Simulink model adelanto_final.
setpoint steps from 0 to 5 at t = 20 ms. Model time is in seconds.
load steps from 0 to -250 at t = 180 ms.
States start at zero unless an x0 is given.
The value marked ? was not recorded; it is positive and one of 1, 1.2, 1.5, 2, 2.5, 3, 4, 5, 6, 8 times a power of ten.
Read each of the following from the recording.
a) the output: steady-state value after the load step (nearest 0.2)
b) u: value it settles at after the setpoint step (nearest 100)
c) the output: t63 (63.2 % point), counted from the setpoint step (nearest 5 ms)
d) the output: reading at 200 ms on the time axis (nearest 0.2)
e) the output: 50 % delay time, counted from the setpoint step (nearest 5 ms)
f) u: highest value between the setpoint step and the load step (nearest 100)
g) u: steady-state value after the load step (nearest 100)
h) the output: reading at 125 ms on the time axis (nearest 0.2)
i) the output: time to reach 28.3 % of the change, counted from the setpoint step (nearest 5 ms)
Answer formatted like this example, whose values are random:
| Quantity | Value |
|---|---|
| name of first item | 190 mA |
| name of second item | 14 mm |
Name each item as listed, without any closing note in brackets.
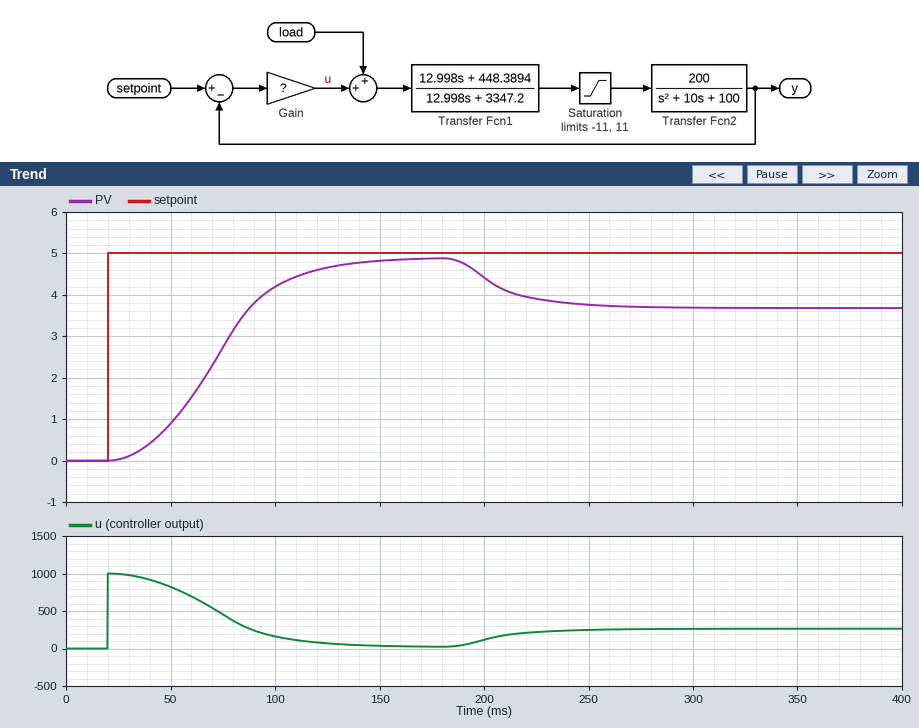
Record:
| Quantity | Value |
|---|---|
| the output: steady-state value after the load step | 3.6 |
| u: value it settles at after the setpoint step | 0 |
| the output: t63 (63.2 % point), counted from the setpoint step | 60 ms |
| the output: reading at 200 ms on the time axis | 4.4 |
| the output: 50 % delay time, counted from the setpoint step | 50 ms |
| u: highest value between the setpoint step and the load step | 1000 |
| u: steady-state value after the load step | 300 |
| the output: reading at 125 ms on the time axis | 4.6 |
| the output: time to reach 28.3 % of the change, counted from the setpoint step | 40 ms |
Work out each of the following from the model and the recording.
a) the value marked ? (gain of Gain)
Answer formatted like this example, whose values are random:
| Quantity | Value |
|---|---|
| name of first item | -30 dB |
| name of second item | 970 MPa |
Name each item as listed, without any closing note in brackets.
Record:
| Quantity | Value |
|---|---|
| the value marked ? | 200 |
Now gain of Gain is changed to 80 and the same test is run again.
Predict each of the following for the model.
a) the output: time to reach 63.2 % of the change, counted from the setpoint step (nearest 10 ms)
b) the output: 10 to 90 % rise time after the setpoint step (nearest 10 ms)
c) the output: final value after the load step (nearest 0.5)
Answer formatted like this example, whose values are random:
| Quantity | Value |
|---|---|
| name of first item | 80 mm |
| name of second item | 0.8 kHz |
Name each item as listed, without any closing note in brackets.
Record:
| Quantity | Value |
|---|---|
| the output: time to reach 63.2 % of the change, counted from the setpoint step | 60 ms |
| the output: 10 to 90 % rise time after the setpoint step | 60 ms |
| the output: final value after the load step | 2.0 |
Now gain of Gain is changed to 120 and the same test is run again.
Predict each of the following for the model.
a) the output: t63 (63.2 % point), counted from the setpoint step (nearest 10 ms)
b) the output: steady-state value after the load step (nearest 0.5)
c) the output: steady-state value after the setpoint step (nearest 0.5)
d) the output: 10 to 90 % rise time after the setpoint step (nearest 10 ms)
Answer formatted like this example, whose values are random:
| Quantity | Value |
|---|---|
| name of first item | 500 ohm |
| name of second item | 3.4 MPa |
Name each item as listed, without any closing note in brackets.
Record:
| Quantity | Value |
|---|---|
| the output: t63 (63.2 % point), counted from the setpoint step | 60 ms |
| the output: steady-state value after the load step | 3.0 |
| the output: steady-state value after the setpoint step | 5.0 |
| the output: 10 to 90 % rise time after the setpoint step | 60 ms |
